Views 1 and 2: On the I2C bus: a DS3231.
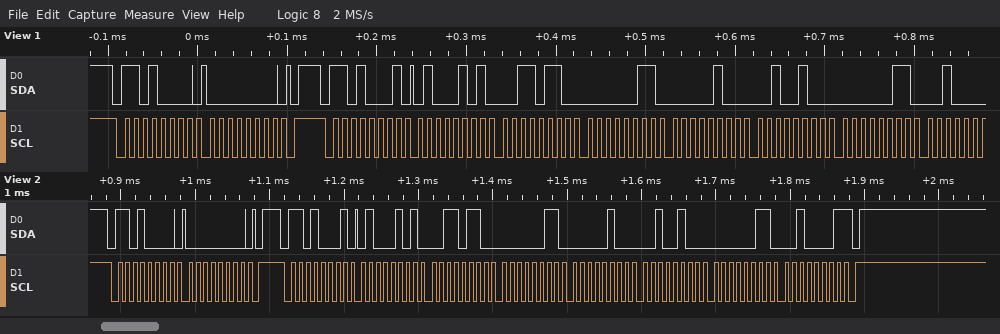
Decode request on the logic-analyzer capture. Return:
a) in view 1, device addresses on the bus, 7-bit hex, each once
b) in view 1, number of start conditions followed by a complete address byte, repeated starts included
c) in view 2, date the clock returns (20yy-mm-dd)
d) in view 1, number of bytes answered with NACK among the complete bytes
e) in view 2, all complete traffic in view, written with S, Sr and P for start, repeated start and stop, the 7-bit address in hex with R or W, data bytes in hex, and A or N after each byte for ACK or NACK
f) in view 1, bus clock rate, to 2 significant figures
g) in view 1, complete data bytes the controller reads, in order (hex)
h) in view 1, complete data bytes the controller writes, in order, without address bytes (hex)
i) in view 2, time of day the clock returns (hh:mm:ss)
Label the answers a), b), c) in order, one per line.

a) 0x68
b) 2
c) 2021-03-24
d) 0
e) S 68W A 00 A P S 68R A 45 A 36 A 03 A 04 A 24 A 03 A 21 N P
f) 100 kHz
g) 45 36 03 04 24 03
h) 00
i) 03:36:45
